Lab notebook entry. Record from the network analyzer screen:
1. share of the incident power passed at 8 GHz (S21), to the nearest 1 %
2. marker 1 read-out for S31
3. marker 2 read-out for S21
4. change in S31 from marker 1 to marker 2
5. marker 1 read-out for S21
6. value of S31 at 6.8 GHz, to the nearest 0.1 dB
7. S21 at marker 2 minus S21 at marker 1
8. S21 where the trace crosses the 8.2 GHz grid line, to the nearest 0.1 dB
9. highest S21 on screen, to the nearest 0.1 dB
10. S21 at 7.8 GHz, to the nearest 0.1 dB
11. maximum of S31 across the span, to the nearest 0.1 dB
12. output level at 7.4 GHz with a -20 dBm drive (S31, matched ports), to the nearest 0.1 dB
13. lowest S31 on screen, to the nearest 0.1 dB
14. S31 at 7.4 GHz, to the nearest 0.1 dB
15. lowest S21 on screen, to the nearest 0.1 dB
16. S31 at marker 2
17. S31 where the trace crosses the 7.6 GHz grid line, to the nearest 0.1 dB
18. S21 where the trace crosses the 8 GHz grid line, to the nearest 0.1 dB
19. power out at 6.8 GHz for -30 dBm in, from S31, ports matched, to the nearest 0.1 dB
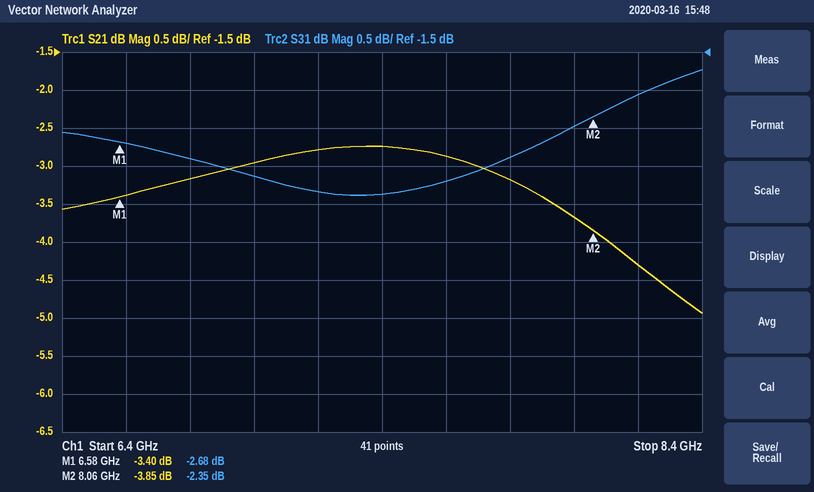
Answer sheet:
43 %
-2.68 dB
-3.85 dB
0.33 dB
-3.40 dB
-2.9 dB
-0.45 dB
-4.3 dB
-2.7 dB
-3.2 dB
-1.7 dB
-23.4 dBm
-3.4 dB
-3.4 dB
-4.9 dB
-2.35 dB
-3.2 dB
-3.7 dB
-32.9 dBm
